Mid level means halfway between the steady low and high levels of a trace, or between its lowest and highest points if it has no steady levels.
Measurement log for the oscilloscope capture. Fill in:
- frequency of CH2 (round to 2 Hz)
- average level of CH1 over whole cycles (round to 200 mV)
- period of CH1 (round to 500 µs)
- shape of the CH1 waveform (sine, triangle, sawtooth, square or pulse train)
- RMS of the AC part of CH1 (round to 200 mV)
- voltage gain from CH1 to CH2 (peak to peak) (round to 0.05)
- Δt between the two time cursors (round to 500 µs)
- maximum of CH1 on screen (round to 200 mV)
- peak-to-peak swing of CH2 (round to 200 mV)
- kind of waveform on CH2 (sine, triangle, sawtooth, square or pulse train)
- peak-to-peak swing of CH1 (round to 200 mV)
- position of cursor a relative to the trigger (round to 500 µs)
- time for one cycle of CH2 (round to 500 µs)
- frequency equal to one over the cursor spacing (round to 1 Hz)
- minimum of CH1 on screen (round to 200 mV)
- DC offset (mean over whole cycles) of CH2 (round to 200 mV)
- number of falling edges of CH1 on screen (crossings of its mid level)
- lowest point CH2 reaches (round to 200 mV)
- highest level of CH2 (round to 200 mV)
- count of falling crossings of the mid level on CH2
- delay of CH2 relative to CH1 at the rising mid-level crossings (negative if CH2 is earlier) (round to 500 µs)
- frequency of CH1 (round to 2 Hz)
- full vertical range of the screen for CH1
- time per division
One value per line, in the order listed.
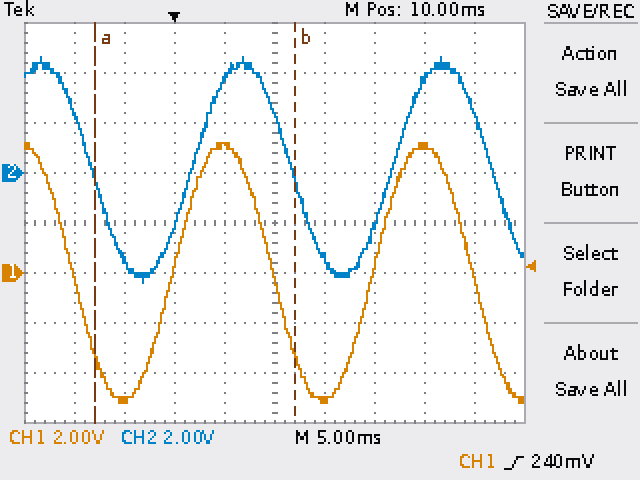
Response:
50 Hz
0.0 V
20.0 ms
sine
3.6 V
0.85
20.0 ms
5.2 V
9.0 V
sine
10.4 V
-8.0 ms
20.0 ms
50 Hz
-5.2 V
200 mV
3
-4.4 V
4.6 V
3
+2.0 ms
50 Hz
16 V
5 ms
